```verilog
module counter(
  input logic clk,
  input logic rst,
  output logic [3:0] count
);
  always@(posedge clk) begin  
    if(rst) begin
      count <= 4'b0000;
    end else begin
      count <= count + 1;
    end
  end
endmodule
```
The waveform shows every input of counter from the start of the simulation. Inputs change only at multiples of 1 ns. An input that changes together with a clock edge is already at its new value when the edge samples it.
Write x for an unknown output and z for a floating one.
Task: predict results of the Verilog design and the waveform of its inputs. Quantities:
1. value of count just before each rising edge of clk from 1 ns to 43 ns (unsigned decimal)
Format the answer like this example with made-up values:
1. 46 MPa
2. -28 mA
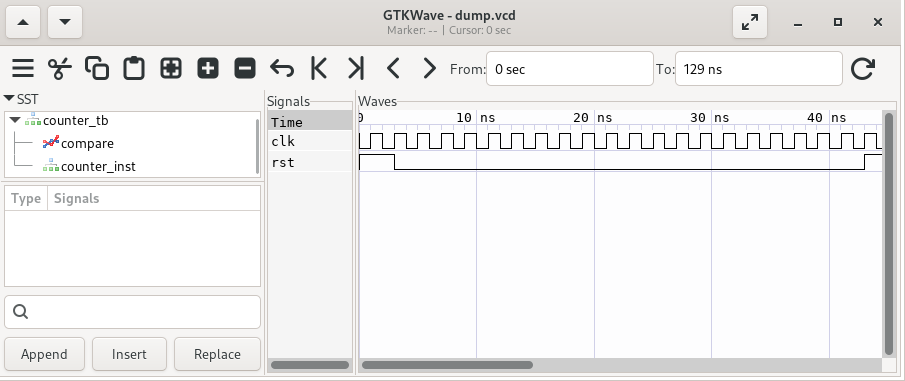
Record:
1. x, 0, 1, 2, 3, 4, 5, 6, 7, 8, 9, 10, 11, 12, 13, 14, 15, 0, 1, 2, 3, 4
